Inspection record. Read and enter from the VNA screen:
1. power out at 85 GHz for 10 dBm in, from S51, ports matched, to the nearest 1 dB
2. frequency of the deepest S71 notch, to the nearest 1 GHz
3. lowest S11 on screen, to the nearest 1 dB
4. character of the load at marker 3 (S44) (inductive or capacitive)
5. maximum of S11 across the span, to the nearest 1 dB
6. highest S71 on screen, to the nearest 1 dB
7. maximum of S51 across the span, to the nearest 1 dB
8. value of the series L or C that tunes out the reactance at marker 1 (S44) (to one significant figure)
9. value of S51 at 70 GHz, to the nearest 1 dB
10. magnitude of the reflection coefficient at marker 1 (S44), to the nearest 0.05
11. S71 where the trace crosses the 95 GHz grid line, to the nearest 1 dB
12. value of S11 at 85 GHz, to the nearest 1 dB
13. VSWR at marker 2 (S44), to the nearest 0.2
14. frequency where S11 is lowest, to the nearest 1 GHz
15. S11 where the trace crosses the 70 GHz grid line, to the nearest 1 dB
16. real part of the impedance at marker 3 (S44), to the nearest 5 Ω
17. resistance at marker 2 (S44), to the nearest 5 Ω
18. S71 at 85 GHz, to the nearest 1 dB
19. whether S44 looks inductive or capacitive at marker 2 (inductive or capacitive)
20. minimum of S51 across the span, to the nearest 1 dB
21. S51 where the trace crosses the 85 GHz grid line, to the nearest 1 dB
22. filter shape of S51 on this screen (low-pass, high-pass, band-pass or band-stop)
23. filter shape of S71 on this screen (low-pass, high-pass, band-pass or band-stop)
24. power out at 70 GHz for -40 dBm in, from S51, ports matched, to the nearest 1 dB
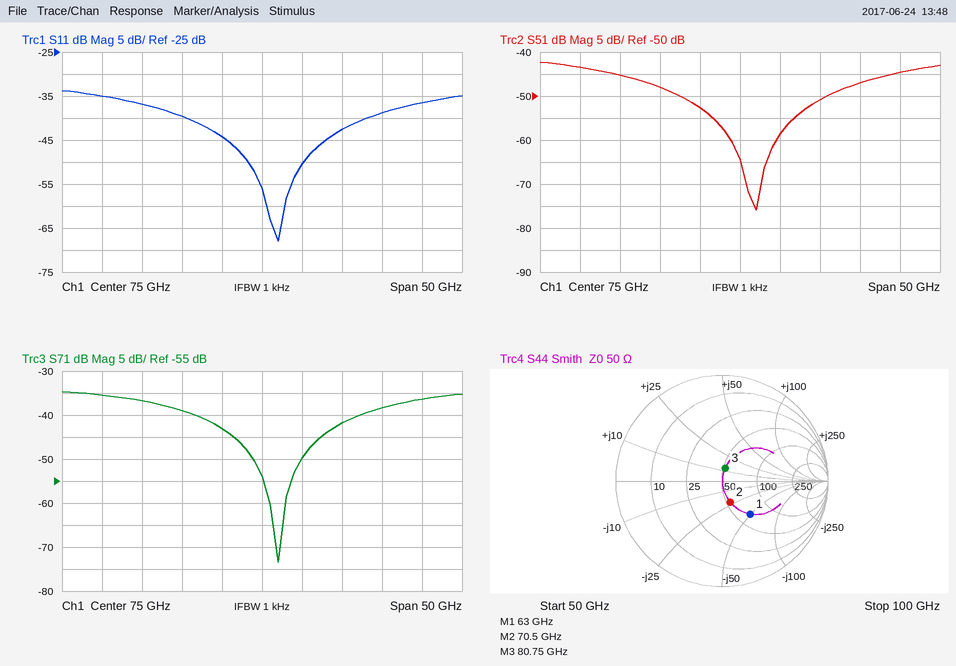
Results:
-41 dBm
77 GHz
-68 dB
inductive
-34 dB
-35 dB
-42 dB
100 pH
-53 dB
0.40
-36 dB
-43 dB
1.6
77 GHz
-44 dB
50 Ω
55 Ω
-42 dB
capacitive
-76 dB
-51 dB
band-stop
band-stop
-93 dBm
